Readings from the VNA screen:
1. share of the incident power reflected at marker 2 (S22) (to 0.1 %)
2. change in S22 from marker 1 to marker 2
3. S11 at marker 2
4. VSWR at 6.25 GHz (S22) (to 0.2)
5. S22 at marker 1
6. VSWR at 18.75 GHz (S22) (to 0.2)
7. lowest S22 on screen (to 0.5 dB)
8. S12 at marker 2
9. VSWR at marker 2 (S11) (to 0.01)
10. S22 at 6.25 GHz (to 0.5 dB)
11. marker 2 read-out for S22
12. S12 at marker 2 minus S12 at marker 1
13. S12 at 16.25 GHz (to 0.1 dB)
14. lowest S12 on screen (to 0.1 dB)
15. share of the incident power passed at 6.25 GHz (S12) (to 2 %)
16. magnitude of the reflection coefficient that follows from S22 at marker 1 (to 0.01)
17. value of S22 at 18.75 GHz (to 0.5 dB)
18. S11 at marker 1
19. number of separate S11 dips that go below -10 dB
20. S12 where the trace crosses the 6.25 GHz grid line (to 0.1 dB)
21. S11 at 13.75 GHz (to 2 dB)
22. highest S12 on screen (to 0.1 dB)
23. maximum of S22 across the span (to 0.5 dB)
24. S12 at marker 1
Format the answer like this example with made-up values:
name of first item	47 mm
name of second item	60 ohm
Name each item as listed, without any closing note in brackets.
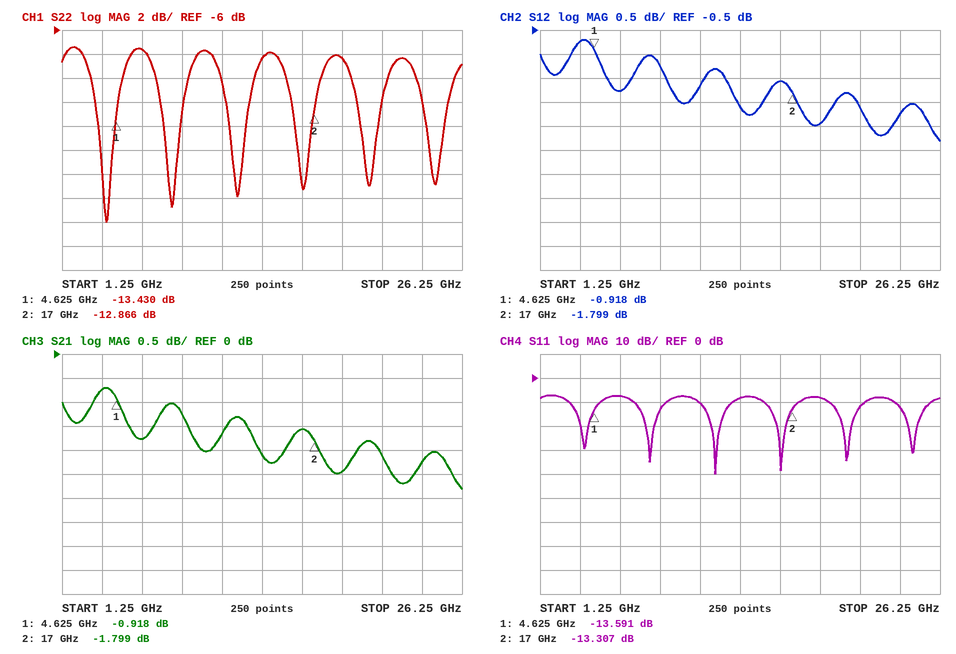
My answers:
share of the incident power reflected at marker 2 (S22)	5.2 %
change in S22 from marker 1 to marker 2	0.564 dB
S11 at marker 2	-13.307 dB
VSWR at 6.25 GHz (S22)	2.4
S22 at marker 1	-13.430 dB
VSWR at 18.75 GHz (S22)	2.2
lowest S22 on screen	-22.0 dB
S12 at marker 2	-1.799 dB
VSWR at marker 2 (S11)	1.55
S22 at 6.25 GHz	-7.5 dB
marker 2 read-out for S22	-12.866 dB
S12 at marker 2 minus S12 at marker 1	-0.881 dB
S12 at 16.25 GHz	-1.6 dB
lowest S12 on screen	-2.8 dB
share of the incident power passed at 6.25 GHz (S12)	66 %
magnitude of the reflection coefficient that follows from S22 at marker 1	0.21
value of S22 at 18.75 GHz	-8.5 dB
S11 at marker 1	-13.591 dB
number of separate S11 dips that go below -10 dB	6
S12 where the trace crosses the 6.25 GHz grid line	-1.8 dB
S11 at 13.75 GHz	-8 dB
highest S12 on screen	-0.7 dB
maximum of S22 across the span	-7.5 dB
S12 at marker 1	-0.918 dB
